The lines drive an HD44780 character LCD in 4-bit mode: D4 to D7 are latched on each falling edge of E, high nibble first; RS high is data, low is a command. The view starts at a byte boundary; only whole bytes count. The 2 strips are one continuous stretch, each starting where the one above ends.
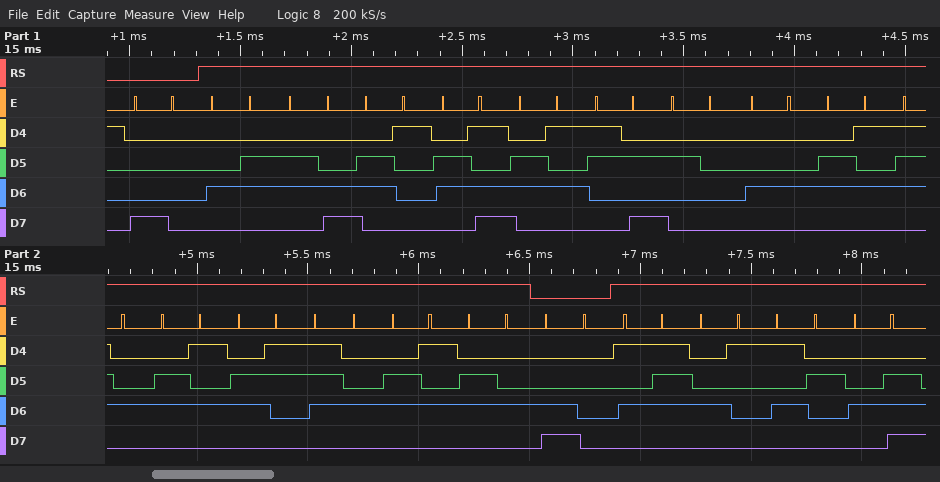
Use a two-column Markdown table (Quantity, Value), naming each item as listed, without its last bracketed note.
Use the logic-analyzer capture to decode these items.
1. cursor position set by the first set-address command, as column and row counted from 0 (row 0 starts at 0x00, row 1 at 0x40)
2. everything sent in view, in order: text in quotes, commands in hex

| Quantity | Value |
|---|---|
| cursor position set by the first set-address command, as column and row counted from 0 | column 0, row 0 |
| everything sent in view, in order: text in quotes, commands in hex | 0x80 "Flame: Detected" 0xC0 "WARN" |
